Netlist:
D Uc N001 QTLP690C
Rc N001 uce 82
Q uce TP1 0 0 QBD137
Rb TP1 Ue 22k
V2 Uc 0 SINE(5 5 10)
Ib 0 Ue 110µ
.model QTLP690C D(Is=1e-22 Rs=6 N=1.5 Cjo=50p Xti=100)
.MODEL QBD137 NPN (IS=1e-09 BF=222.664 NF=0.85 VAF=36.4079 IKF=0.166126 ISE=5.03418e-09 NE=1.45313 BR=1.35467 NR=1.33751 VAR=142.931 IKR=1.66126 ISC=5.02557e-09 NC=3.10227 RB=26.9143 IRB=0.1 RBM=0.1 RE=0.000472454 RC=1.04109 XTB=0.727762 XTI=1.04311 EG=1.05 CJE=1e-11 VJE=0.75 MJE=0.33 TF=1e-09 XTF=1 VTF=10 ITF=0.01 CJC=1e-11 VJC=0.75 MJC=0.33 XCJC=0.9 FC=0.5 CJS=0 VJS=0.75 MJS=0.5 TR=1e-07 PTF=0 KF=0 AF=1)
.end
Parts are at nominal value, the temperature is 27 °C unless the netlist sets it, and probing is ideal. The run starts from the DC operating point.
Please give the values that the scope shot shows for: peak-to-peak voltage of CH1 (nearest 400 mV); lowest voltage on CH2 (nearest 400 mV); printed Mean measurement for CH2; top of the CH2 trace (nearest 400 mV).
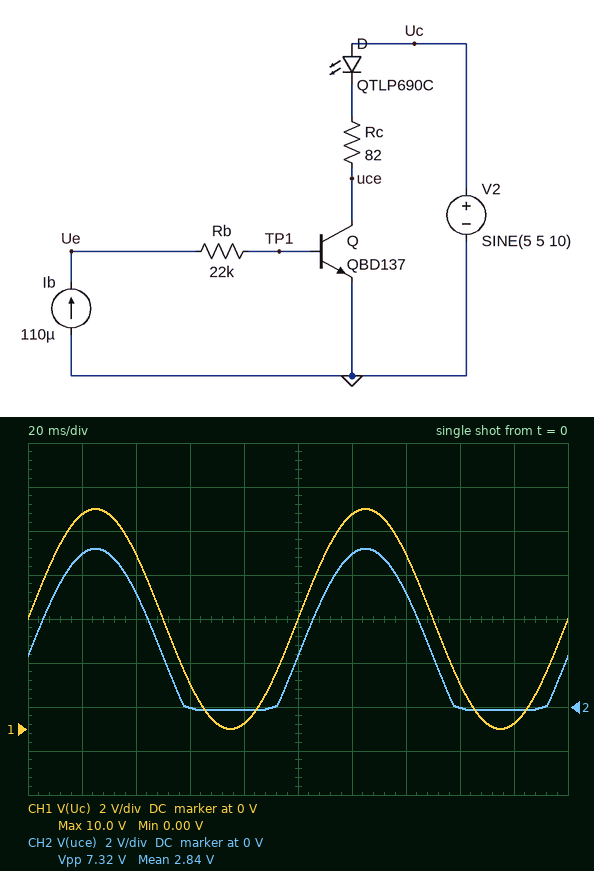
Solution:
10.0 V
0 V
2.84 V
7.2 V
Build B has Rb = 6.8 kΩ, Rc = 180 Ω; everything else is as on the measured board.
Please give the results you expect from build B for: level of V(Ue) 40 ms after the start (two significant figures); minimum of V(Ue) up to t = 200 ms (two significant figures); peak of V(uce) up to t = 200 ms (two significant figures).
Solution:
1.1 V
1.0 V
6.1 V
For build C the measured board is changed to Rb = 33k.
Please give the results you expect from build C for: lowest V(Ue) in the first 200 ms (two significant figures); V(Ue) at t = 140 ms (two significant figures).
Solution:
3.9 V
4.0 V
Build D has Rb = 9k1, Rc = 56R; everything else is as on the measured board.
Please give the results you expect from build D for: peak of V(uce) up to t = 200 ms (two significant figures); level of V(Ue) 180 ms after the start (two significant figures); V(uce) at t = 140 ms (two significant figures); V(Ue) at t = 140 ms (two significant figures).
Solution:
7.5 V
1.3 V
5.5 V
1.4 V
